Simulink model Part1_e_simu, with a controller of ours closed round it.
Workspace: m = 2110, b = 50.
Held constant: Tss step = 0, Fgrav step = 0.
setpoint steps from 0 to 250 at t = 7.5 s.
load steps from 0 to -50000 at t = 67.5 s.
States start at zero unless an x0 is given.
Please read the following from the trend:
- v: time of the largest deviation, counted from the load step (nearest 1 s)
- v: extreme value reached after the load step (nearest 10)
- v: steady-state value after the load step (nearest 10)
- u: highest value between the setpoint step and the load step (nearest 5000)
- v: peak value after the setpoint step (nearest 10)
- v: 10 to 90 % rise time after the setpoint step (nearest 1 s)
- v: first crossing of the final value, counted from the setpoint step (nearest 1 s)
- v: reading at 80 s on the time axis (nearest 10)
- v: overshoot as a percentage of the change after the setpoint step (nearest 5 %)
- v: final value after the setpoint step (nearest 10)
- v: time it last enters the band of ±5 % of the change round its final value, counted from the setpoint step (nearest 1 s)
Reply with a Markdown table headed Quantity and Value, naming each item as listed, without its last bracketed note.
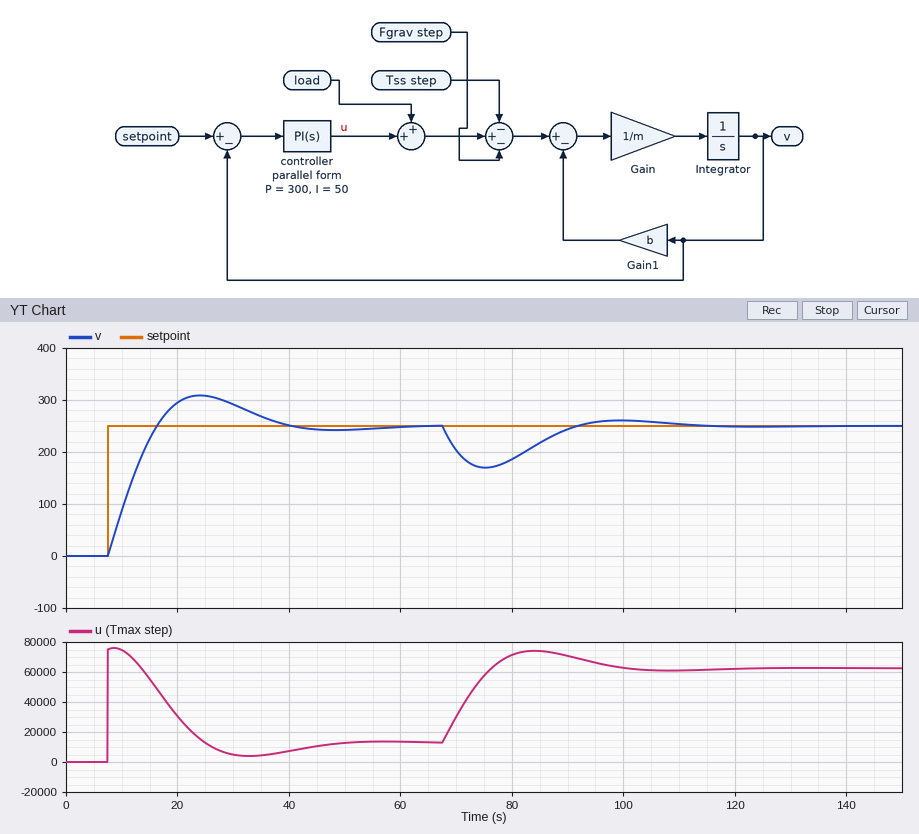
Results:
| Quantity | Value |
|---|---|
| v: time of the largest deviation, counted from the load step | 8 s |
| v: extreme value reached after the load step | 170 |
| v: steady-state value after the load step | 250 |
| u: highest value between the setpoint step and the load step | 75000 |
| v: peak value after the setpoint step | 310 |
| v: 10 to 90 % rise time after the setpoint step | 7 s |
| v: first crossing of the final value, counted from the setpoint step | 9 s |
| v: reading at 80 s on the time axis | 190 |
| v: overshoot as a percentage of the change after the setpoint step | 25 % |
| v: final value after the setpoint step | 250 |
| v: time it last enters the band of ±5 % of the change round its final value, counted from the setpoint step | 29 s |
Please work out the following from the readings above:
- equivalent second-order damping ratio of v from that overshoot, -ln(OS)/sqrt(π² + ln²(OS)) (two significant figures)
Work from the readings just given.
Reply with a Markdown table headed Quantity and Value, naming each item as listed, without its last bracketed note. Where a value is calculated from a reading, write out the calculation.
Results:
| Quantity | Value |
|---|---|
| equivalent second-order damping ratio of v from that overshoot, -ln(OS)/sqrt(π² + ln²(OS)) | ln(0.25) = -1.386; 1.386 / sqrt(9.870 + 1.922) = 0.40 |
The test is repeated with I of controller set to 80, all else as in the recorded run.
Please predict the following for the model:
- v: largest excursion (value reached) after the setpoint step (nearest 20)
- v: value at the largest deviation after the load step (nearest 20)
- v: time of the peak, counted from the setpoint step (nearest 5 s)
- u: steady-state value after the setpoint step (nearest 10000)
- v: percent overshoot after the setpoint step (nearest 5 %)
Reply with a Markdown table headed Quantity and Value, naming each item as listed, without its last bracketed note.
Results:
| Quantity | Value |
|---|---|
| v: largest excursion (value reached) after the setpoint step | 320 |
| v: value at the largest deviation after the load step | 180 |
| v: time of the peak, counted from the setpoint step | 15 s |
| u: steady-state value after the setpoint step | 10000 |
| v: percent overshoot after the setpoint step | 30 % |
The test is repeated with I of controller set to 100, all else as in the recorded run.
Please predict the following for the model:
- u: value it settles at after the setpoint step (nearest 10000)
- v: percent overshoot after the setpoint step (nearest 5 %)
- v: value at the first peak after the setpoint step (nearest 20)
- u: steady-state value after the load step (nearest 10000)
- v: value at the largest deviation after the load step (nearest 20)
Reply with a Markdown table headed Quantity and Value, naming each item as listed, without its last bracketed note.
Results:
| Quantity | Value |
|---|---|
| u: value it settles at after the setpoint step | 10000 |
| v: percent overshoot after the setpoint step | 35 % |
| v: value at the first peak after the setpoint step | 340 |
| u: steady-state value after the load step | 60000 |
| v: value at the largest deviation after the load step | 180 |
